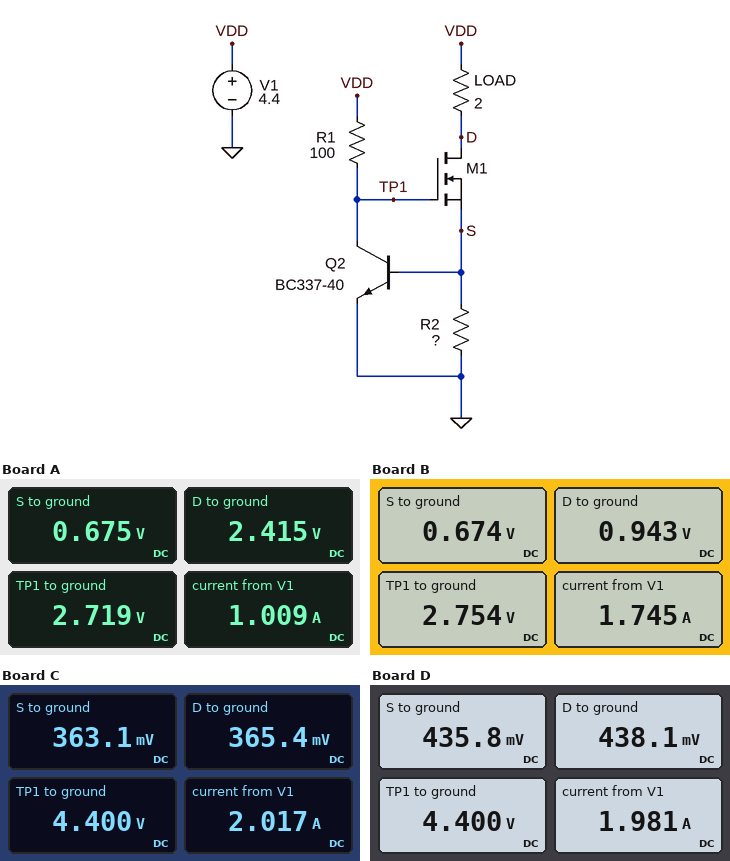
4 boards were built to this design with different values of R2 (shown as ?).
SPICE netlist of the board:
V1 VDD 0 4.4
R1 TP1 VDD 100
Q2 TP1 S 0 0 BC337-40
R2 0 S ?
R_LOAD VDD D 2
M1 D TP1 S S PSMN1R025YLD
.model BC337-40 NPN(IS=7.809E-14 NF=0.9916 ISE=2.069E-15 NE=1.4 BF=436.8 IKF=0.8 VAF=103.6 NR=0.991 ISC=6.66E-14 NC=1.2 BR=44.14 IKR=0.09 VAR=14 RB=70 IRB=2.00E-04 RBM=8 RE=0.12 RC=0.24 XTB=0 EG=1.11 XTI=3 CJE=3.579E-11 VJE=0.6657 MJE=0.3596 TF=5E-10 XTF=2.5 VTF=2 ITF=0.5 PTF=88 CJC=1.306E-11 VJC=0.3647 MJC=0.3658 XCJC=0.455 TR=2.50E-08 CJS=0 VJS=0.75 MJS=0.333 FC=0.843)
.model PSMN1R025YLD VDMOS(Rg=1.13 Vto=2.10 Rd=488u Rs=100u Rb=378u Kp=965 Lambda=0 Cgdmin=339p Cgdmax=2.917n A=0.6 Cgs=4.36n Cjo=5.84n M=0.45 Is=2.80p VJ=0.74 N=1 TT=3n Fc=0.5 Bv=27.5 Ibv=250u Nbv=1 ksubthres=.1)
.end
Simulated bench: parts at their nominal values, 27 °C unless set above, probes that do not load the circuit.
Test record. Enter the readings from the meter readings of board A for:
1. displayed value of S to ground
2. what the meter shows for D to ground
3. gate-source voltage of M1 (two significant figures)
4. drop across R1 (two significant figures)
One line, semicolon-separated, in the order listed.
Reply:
0.675 V; 2.415 V; 2.0 V; 1.7 V
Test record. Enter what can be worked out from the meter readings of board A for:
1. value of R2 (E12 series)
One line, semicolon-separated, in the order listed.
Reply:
0.68 Ω
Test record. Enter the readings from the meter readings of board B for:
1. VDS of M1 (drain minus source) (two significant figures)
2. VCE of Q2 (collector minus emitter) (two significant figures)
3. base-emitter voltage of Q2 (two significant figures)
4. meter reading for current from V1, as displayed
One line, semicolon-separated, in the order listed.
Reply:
270 mV; 2.8 V; 670 mV; 1.745 A
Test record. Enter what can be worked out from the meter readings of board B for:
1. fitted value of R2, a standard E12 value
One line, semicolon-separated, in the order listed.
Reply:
0.39 Ω
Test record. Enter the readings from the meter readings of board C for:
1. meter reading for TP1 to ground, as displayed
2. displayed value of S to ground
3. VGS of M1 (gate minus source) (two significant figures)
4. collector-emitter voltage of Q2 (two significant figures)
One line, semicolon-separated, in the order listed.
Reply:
4.400 V; 363.1 mV; 4.0 V; 4.4 V
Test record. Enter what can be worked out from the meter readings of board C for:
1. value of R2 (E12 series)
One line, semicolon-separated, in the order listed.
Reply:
0.18 Ω
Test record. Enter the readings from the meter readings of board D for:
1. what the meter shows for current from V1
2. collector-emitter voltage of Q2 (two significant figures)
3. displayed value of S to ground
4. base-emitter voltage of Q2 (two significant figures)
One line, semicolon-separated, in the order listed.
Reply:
1.981 A; 4.4 V; 435.8 mV; 440 mV
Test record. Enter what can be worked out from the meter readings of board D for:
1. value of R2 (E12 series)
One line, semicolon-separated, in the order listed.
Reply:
0.22 Ω
